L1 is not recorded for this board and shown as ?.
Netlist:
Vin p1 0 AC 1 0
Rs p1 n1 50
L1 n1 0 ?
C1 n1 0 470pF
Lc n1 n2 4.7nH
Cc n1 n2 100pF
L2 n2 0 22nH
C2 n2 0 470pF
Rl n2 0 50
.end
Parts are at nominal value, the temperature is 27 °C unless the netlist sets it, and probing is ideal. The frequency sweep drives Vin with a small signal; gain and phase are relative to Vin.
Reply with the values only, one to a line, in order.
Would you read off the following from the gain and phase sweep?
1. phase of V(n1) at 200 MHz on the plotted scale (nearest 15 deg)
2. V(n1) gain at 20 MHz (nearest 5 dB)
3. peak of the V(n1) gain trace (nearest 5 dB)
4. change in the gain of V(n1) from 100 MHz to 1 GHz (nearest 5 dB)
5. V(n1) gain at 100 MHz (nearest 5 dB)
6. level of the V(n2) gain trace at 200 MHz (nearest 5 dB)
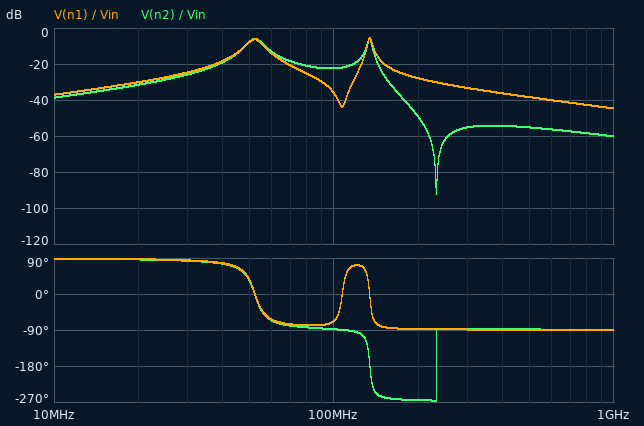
-90 deg
-30 dB
-5 dB
-10 dB
-35 dB
-50 dB
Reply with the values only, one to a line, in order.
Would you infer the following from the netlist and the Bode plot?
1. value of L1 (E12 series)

18 nH
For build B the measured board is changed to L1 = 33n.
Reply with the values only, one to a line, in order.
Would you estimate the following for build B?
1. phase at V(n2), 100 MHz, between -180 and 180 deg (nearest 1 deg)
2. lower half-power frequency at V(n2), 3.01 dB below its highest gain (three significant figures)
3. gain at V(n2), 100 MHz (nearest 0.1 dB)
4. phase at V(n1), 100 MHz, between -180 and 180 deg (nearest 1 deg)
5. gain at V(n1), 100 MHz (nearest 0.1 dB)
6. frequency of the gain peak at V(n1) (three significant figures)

-89 deg
41.9 MHz
-22.7 dB
-68 deg
-36.4 dB
45.1 MHz
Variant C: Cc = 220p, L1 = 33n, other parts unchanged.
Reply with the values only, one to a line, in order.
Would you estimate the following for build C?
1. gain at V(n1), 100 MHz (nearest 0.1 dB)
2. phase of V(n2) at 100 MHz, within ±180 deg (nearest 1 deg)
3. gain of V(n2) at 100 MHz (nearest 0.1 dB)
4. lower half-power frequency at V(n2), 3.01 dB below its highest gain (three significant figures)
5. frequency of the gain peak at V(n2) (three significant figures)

-36.3 dB
-92 deg
-19.9 dB
41.9 MHz
45.1 MHz
